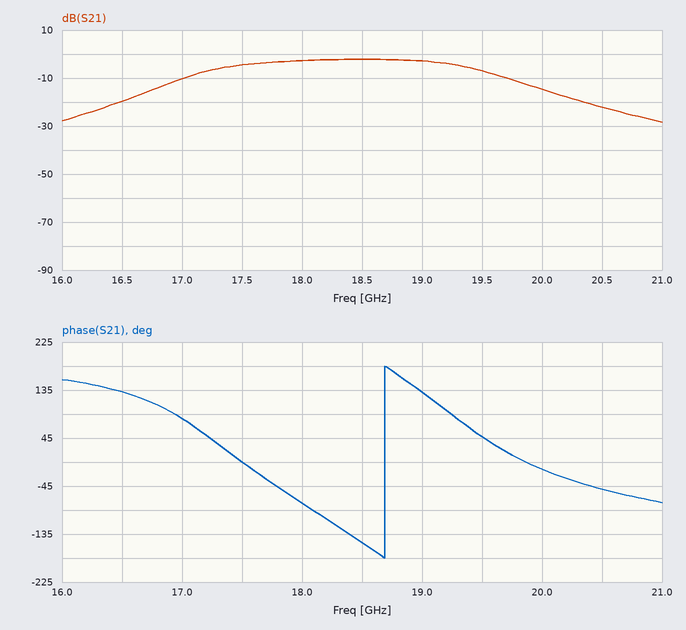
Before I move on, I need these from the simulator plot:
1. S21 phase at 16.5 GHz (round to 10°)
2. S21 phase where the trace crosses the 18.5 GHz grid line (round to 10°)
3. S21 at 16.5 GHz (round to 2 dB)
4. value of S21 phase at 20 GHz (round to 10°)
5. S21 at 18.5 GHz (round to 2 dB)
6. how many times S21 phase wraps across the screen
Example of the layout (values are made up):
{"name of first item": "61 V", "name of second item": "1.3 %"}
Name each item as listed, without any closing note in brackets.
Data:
{"S21 phase at 16.5 GHz": "130°", "S21 phase where the trace crosses the 18.5 GHz grid line": "-150°", "S21 at 16.5 GHz": "-20 dB", "value of S21 phase at 20 GHz": "-10°", "S21 at 18.5 GHz": "-2 dB", "how many times S21 phase wraps across the screen": "1"}
